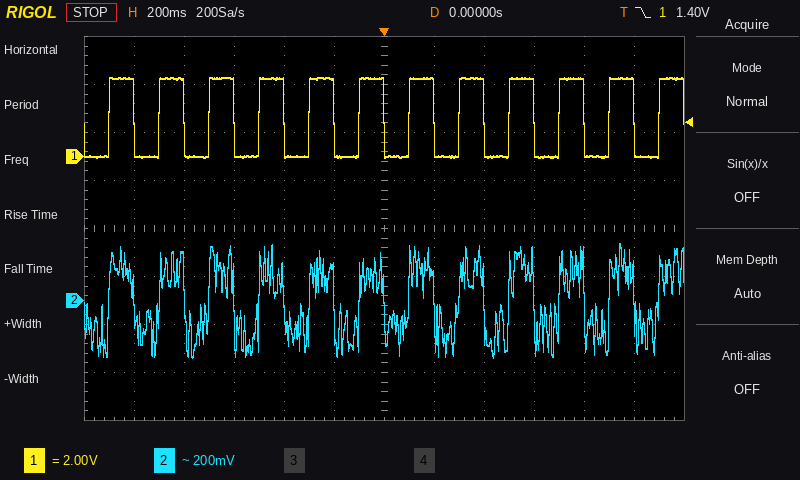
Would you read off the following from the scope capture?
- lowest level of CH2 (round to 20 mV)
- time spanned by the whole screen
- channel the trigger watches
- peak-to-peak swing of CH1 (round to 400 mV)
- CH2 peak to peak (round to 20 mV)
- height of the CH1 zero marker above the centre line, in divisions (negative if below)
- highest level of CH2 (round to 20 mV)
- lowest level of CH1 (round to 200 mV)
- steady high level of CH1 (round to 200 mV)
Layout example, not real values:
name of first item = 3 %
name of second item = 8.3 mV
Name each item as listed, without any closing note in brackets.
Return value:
lowest level of CH2 = -240 mV
time spanned by the whole screen = 2.4 s
channel the trigger watches = CH1
peak-to-peak swing of CH1 = 3.2 V
CH2 peak to peak = 480 mV
height of the CH1 zero marker above the centre line, in divisions = +1.5 div
highest level of CH2 = 240 mV
lowest level of CH1 = 0.0 V
steady high level of CH1 = 3.2 V
